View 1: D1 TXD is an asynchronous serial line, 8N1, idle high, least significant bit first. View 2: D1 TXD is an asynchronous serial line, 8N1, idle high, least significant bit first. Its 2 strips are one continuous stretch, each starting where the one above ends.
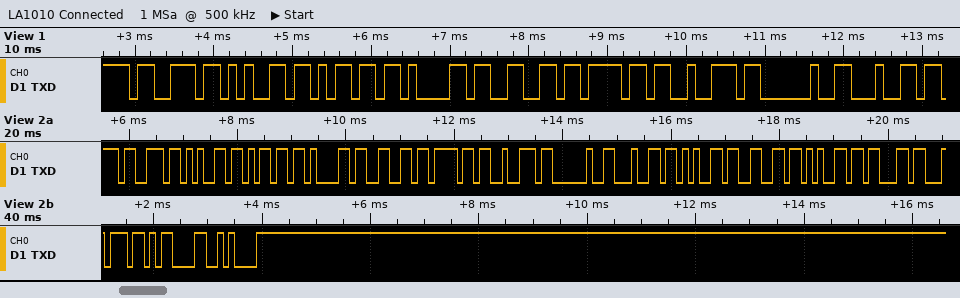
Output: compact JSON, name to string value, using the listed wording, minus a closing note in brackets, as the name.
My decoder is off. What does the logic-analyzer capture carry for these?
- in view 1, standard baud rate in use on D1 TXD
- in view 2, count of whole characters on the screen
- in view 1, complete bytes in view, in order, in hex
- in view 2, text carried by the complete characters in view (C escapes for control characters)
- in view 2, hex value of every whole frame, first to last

{"in view 1, standard baud rate in use on D1 TXD": "9600 baud", "in view 2, count of whole characters on the screen": "16", "in view 1, complete bytes in view, in order, in hex": "73 65 6D 61 66 6F 72 20 64", "in view 2, text carried by the complete characters in view": "\"semafor defect\\r\\n\"", "in view 2, hex value of every whole frame, first to last": "73 65 6D 61 66 6F 72 20 64 65 66 65 63 74 0D 0A"}
